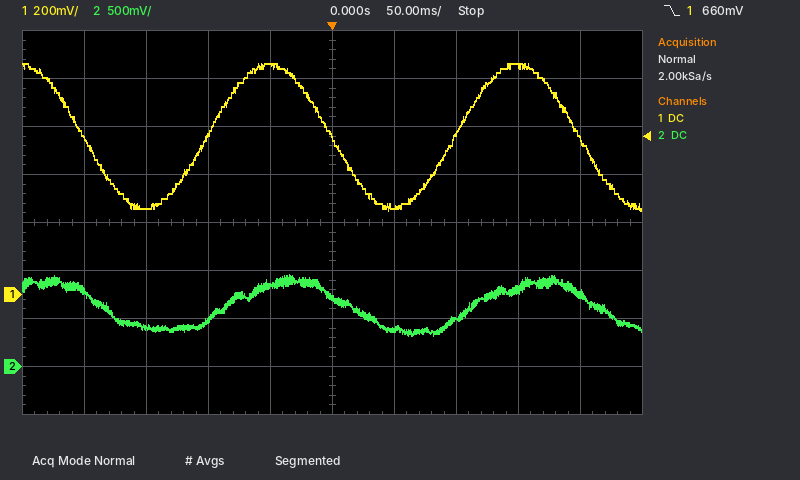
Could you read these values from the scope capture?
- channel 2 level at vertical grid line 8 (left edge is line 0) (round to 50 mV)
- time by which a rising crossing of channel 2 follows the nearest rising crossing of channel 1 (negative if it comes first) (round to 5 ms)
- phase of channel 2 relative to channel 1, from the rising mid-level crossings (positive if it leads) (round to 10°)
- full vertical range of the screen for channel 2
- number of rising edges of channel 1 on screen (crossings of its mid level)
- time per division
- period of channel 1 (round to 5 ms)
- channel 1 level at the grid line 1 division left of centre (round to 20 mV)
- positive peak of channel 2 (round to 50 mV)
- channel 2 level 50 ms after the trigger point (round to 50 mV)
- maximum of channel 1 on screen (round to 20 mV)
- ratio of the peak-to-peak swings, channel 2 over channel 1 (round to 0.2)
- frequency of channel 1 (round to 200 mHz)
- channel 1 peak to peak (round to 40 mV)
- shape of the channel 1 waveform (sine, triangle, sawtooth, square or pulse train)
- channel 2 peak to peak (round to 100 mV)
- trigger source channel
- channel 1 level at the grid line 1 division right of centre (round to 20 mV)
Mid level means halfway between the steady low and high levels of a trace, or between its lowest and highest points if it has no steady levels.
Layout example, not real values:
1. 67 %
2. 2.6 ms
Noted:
1. 800 mV
2. +15 ms
3. -30°
4. 4 V
5. 2
6. 50 ms
7. 200 ms
8. 960 mV
9. 950 mV
10. 400 mV
11. 960 mV
12. 1.0
13. 5.0 Hz
14. 600 mV
15. sine
16. 600 mV
17. channel 1
18. 360 mV
